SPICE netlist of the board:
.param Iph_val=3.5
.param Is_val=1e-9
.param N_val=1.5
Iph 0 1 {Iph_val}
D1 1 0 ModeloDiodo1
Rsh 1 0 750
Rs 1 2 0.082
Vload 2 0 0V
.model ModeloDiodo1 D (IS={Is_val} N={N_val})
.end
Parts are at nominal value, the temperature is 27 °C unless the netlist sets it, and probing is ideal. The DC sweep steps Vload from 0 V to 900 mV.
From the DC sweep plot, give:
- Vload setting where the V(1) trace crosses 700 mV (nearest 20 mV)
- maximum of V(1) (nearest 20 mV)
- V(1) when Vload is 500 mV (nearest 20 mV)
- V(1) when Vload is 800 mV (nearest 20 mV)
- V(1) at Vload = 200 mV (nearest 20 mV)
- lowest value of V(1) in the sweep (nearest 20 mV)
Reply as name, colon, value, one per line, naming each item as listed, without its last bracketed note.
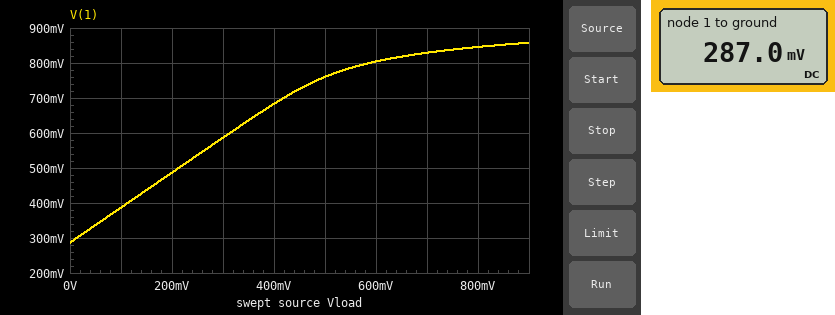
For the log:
Vload setting where the V(1) trace crosses 700 mV: 420 mV
maximum of V(1): 860 mV
V(1) when Vload is 500 mV: 760 mV
V(1) when Vload is 800 mV: 840 mV
V(1) at Vload = 200 mV: 480 mV
lowest value of V(1) in the sweep: 280 mV
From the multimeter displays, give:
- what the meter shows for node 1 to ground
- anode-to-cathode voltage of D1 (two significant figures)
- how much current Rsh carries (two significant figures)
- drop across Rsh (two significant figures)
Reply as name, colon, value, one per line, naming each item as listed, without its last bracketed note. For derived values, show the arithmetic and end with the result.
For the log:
what the meter shows for node 1 to ground: 287.0 mV
anode-to-cathode voltage of D1: 287 mV = 290 mV
how much current Rsh carries: (287 mV) / 750 Ω = 380 µA
drop across Rsh: 287 mV = 290 mV
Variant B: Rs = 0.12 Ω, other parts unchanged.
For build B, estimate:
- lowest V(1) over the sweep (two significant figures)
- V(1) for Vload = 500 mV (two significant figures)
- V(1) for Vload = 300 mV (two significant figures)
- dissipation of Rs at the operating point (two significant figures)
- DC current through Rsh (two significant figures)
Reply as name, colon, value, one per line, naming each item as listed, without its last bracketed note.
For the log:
lowest V(1) over the sweep: 420 mV
V(1) for Vload = 500 mV: 800 mV
V(1) for Vload = 300 mV: 710 mV
dissipation of Rs at the operating point: 1.5 W
DC current through Rsh: 560 µA
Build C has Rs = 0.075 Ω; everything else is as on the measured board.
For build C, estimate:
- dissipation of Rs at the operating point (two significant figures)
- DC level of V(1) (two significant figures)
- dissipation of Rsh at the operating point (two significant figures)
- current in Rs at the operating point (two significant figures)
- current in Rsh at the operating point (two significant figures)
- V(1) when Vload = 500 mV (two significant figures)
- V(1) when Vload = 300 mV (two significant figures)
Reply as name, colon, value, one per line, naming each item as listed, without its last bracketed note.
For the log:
dissipation of Rs at the operating point: 920 mW
DC level of V(1): 260 mV
dissipation of Rsh at the operating point: 92 µW
current in Rs at the operating point: 3.5 A
current in Rsh at the operating point: 350 µA
V(1) when Vload = 500 mV: 750 mV
V(1) when Vload = 300 mV: 560 mV
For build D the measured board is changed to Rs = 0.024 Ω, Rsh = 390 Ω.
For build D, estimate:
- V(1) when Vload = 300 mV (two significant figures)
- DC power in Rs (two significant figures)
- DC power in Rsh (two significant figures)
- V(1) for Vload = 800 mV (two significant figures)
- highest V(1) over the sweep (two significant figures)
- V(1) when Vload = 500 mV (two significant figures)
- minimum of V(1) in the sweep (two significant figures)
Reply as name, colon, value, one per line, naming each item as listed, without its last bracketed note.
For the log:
V(1) when Vload = 300 mV: 380 mV
DC power in Rs: 290 mW
DC power in Rsh: 18 µW
V(1) for Vload = 800 mV: 830 mV
highest V(1) over the sweep: 870 mV
V(1) when Vload = 500 mV: 580 mV
minimum of V(1) in the sweep: 84 mV
